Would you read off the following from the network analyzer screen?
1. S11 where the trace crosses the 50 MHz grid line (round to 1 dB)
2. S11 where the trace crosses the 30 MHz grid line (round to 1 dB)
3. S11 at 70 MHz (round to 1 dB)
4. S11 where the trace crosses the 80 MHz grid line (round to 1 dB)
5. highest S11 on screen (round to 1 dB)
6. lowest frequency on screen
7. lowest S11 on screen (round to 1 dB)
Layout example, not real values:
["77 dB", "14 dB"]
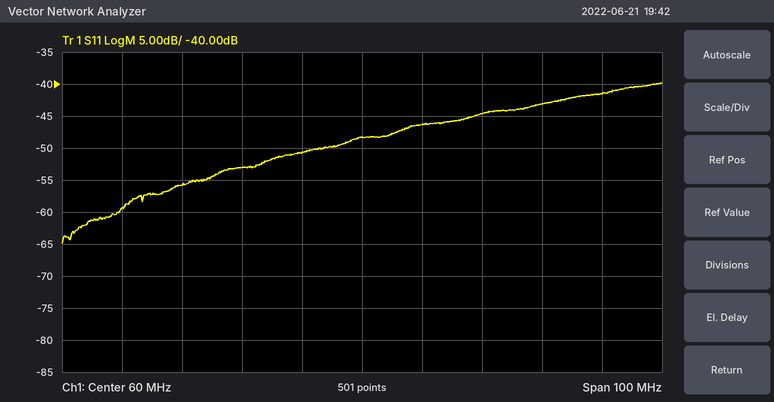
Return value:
["-51 dB", "-56 dB", "-46 dB", "-45 dB", "-40 dB", "10 MHz", "-65 dB"]
